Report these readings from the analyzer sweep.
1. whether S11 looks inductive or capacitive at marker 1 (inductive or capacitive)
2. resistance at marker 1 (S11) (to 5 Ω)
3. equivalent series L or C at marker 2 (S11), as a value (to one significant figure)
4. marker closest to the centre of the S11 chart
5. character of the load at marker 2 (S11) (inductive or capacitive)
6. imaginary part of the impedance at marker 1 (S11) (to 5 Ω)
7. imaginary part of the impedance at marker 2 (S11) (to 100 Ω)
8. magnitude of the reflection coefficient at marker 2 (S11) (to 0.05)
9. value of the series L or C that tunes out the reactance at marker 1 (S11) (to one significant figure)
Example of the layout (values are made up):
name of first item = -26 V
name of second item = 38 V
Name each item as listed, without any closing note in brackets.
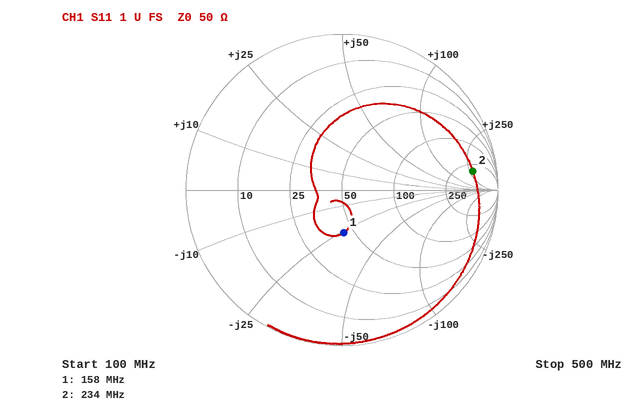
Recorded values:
whether S11 looks inductive or capacitive at marker 1 = capacitive
resistance at marker 1 (S11) = 45 Ω
equivalent series L or C at marker 2 (S11), as a value = 200 nH
marker closest to the centre of the S11 chart = marker 1
character of the load at marker 2 (S11) = inductive
imaginary part of the impedance at marker 1 (S11) = -25 Ω
imaginary part of the impedance at marker 2 (S11) = +300 Ω
magnitude of the reflection coefficient at marker 2 (S11) = 0.85
value of the series L or C that tunes out the reactance at marker 1 (S11) = 30 nH
